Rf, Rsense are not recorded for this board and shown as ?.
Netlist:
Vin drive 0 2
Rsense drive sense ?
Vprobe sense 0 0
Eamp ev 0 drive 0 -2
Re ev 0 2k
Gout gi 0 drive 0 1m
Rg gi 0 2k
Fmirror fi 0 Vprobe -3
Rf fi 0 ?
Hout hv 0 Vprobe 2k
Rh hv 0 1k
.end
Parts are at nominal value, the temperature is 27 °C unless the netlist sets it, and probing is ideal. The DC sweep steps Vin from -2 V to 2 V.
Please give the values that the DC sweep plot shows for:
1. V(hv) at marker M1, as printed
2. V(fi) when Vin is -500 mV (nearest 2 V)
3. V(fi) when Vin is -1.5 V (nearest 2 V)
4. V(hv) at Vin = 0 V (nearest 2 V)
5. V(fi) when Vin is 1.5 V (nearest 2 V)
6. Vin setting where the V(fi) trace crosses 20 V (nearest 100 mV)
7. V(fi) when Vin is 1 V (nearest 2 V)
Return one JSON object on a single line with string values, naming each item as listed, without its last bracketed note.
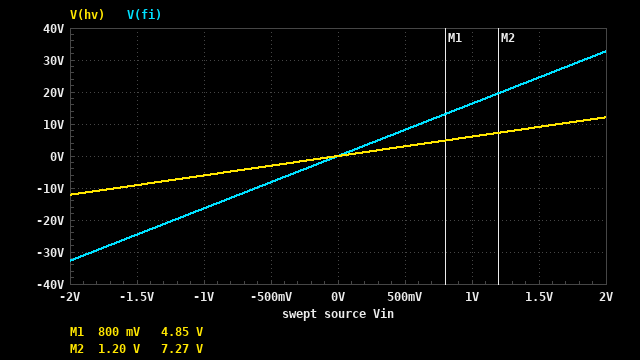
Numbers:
{"V(hv) at marker M1, as printed": "4.85 V", "V(fi) when Vin is -500 mV": "-8 V", "V(fi) when Vin is -1.5 V": "-24 V", "V(hv) at Vin = 0 V": "0 V", "V(fi) when Vin is 1.5 V": "24 V", "Vin setting where the V(fi) trace crosses 20 V": "1.2 V", "V(fi) when Vin is 1 V": "16 V"}
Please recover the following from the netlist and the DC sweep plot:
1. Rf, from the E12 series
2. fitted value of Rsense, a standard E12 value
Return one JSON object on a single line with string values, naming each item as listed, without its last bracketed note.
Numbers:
{"Rf, from the E12 series": "1.8 kΩ", "fitted value of Rsense, a standard E12 value": "330 Ω"}
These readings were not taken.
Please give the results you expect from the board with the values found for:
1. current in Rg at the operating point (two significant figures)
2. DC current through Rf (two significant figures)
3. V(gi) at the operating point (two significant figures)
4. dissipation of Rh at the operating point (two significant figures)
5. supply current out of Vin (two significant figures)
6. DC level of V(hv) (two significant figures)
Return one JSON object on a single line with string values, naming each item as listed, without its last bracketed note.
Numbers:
{"current in Rg at the operating point": "2.0 mA", "DC current through Rf": "18 mA", "V(gi) at the operating point": "-4.0 V", "dissipation of Rh at the operating point": "150 mW", "supply current out of Vin": "6.1 mA", "DC level of V(hv)": "12 V"}
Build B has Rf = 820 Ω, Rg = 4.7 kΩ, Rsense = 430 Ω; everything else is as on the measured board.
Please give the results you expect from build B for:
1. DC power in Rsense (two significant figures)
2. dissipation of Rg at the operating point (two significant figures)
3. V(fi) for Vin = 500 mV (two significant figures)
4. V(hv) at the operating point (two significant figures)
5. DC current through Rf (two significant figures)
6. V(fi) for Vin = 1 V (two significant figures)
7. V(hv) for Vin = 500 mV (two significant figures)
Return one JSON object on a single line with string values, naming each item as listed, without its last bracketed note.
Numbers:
{"DC power in Rsense": "9.3 mW", "dissipation of Rg at the operating point": "19 mW", "V(fi) for Vin = 500 mV": "2.9 V", "V(hv) at the operating point": "9.3 V", "DC current through Rf": "14 mA", "V(fi) for Vin = 1 V": "5.7 V", "V(hv) for Vin = 500 mV": "2.3 V"}
